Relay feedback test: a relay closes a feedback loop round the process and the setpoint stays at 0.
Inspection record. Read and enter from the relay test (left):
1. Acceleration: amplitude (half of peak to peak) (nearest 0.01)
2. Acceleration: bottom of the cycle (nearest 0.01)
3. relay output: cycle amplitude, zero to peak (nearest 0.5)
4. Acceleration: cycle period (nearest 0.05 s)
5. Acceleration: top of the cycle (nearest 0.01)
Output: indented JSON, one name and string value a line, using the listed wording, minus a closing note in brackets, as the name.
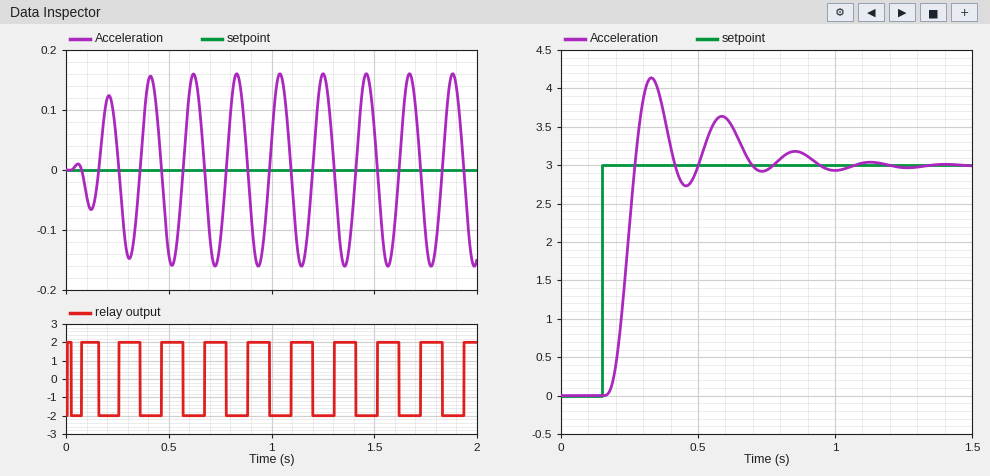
{
  "Acceleration: amplitude (half of peak to peak)": "0.16",
  "Acceleration: bottom of the cycle": "-0.16",
  "relay output: cycle amplitude, zero to peak": "2.0",
  "Acceleration: cycle period": "0.20 s",
  "Acceleration: top of the cycle": "0.16"
}
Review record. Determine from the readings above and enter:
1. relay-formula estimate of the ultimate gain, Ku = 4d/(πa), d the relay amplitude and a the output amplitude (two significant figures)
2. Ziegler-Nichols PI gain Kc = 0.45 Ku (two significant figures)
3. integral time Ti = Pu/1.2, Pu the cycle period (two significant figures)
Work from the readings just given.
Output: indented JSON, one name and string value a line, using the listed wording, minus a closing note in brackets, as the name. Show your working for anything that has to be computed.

{
  "relay-formula estimate of the ultimate gain, Ku = 4d/(πa), d the relay amplitude and a the output amplitude": "4 × 2 / (π × 0.16) = 16",
  "Ziegler-Nichols PI gain Kc = 0.45 Ku": "0.45 × 16 = 7.2",
  "integral time Ti = Pu/1.2, Pu the cycle period": "0.2 / 1.2 = 0.17 s"
}
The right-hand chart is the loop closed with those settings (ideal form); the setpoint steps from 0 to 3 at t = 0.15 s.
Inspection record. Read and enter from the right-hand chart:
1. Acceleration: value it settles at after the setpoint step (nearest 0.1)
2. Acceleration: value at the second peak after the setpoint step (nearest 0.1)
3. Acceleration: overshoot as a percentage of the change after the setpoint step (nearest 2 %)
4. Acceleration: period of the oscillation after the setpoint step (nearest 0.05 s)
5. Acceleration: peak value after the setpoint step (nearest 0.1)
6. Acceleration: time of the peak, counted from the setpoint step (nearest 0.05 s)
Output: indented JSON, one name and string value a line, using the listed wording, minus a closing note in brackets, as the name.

{
  "Acceleration: value it settles at after the setpoint step": "3.0",
  "Acceleration: value at the second peak after the setpoint step": "3.6",
  "Acceleration: overshoot as a percentage of the change after the setpoint step": "38 %",
  "Acceleration: period of the oscillation after the setpoint step": "0.25 s",
  "Acceleration: peak value after the setpoint step": "4.1",
  "Acceleration: time of the peak, counted from the setpoint step": "0.20 s"
}
